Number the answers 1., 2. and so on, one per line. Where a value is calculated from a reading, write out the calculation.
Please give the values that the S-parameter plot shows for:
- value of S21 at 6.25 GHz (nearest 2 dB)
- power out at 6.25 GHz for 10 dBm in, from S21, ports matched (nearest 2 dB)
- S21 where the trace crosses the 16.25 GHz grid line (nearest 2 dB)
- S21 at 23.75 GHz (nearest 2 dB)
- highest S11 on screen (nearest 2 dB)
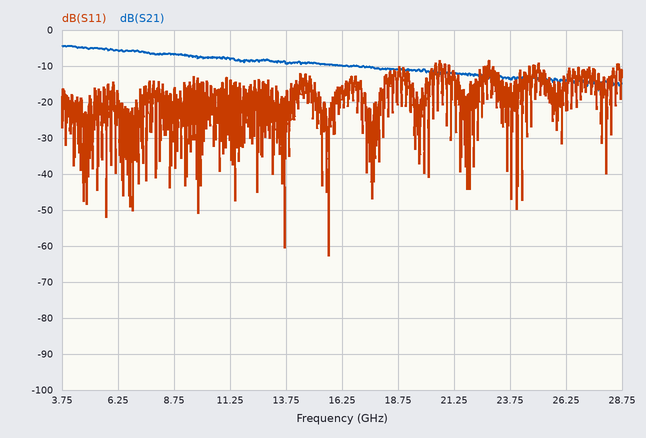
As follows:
1. -6 dB
2. 10 dBm + (-6 dB) = 4 dBm
3. -10 dB
4. -14 dB
5. -8 dB
